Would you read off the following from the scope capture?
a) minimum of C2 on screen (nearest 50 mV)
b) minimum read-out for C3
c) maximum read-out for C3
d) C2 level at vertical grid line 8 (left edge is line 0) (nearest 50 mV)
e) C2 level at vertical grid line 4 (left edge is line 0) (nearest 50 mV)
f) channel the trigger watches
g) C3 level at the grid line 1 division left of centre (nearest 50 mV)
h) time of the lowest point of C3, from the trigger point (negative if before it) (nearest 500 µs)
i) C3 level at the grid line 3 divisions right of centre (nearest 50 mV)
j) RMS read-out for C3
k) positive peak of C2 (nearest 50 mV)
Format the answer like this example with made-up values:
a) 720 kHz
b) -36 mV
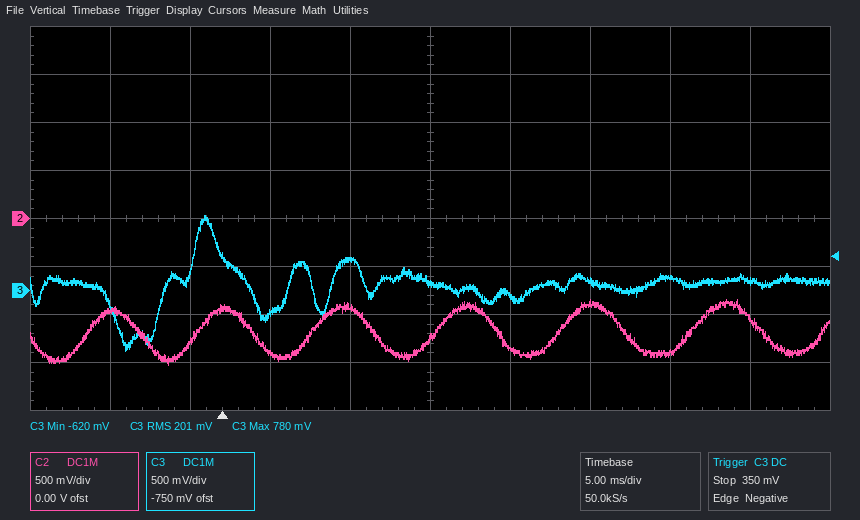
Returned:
a) -1.50 V
b) -620 mV
c) 780 mV
d) -1.40 V
e) -900 mV
f) C3
g) 300 mV
h) -6.0 ms
i) 150 mV
j) 201 mV
k) -850 mV
